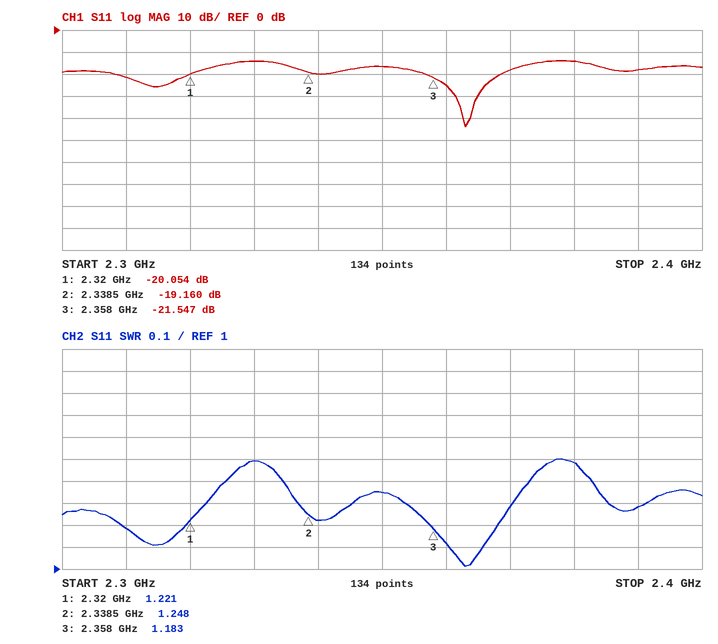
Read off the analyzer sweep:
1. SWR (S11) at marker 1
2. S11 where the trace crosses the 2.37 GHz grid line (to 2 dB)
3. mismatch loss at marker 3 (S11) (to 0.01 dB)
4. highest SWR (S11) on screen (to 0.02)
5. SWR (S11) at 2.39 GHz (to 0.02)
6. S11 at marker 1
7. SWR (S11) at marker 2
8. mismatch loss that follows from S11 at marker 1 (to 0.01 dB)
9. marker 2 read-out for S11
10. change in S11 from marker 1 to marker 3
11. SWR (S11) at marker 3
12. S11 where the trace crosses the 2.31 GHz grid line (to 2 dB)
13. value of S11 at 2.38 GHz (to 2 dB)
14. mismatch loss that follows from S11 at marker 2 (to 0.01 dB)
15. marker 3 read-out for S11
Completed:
1.221
-18 dB
0.03 dB
1.50
1.28
-20.054 dB
1.248
0.04 dB
-19.160 dB
-1.493 dB
1.183
-22 dB
-14 dB
0.05 dB
-21.547 dB
